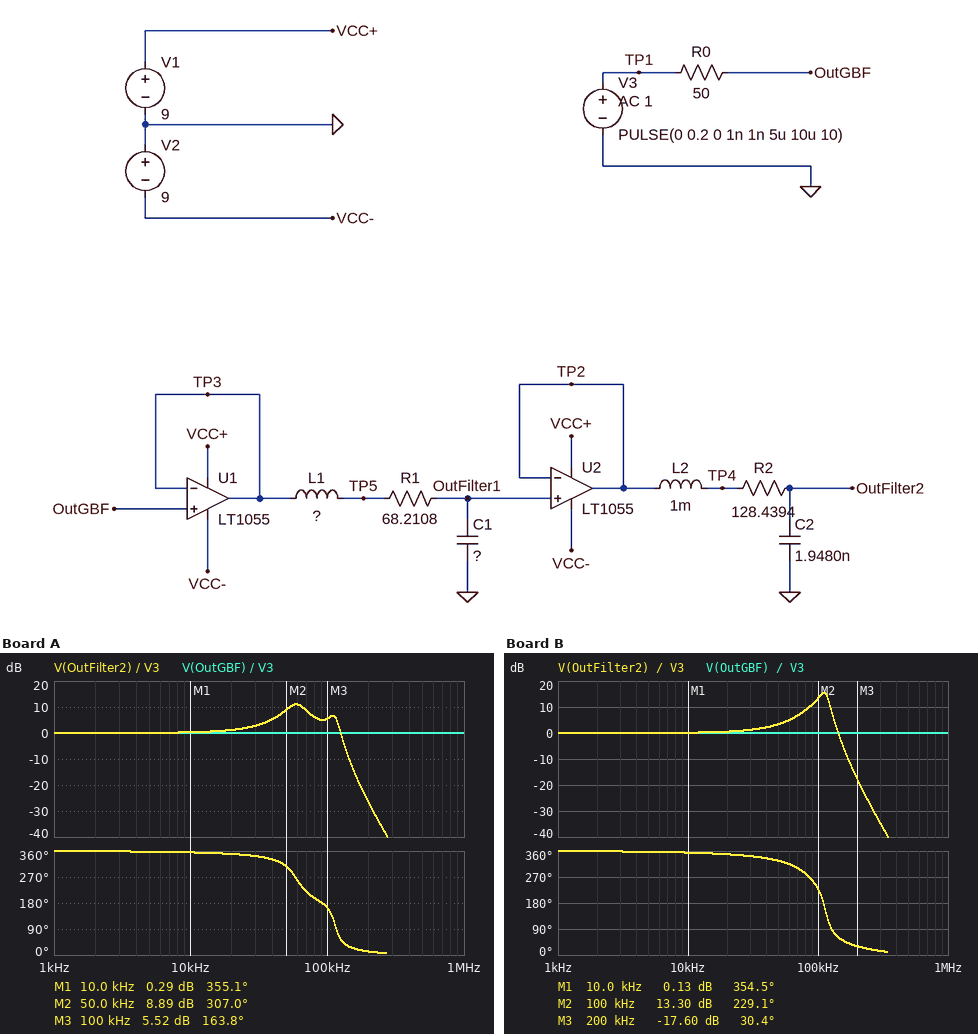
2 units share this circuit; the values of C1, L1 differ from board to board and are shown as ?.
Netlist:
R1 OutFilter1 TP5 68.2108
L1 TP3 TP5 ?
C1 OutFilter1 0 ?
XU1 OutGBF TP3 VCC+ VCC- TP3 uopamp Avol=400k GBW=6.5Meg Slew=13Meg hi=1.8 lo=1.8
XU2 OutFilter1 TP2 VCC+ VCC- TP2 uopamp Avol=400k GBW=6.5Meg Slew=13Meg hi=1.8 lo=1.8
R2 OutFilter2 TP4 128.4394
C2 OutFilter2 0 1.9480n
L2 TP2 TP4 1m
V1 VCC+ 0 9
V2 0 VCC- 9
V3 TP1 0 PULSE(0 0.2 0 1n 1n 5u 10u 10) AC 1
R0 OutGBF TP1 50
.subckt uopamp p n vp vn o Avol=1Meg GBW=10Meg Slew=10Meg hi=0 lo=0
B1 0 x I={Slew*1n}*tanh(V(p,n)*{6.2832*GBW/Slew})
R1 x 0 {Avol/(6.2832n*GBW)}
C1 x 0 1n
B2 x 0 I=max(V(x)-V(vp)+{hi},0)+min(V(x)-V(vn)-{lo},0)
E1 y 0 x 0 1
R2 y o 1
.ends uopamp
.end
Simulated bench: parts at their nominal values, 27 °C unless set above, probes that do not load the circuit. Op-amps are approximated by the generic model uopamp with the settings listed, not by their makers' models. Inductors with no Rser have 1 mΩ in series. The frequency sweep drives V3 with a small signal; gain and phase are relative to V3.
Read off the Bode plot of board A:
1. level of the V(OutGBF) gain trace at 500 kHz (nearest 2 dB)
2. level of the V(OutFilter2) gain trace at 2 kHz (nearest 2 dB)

0 dB
0 dB
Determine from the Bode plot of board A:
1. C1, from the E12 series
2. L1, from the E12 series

15 nF
470 µH
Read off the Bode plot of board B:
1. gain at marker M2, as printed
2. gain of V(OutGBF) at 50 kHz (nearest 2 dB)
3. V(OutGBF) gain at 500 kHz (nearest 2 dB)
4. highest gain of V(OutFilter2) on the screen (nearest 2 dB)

13.30 dB
0 dB
0 dB
16 dB
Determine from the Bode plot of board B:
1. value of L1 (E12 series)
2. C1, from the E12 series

150 µH
18 nF
